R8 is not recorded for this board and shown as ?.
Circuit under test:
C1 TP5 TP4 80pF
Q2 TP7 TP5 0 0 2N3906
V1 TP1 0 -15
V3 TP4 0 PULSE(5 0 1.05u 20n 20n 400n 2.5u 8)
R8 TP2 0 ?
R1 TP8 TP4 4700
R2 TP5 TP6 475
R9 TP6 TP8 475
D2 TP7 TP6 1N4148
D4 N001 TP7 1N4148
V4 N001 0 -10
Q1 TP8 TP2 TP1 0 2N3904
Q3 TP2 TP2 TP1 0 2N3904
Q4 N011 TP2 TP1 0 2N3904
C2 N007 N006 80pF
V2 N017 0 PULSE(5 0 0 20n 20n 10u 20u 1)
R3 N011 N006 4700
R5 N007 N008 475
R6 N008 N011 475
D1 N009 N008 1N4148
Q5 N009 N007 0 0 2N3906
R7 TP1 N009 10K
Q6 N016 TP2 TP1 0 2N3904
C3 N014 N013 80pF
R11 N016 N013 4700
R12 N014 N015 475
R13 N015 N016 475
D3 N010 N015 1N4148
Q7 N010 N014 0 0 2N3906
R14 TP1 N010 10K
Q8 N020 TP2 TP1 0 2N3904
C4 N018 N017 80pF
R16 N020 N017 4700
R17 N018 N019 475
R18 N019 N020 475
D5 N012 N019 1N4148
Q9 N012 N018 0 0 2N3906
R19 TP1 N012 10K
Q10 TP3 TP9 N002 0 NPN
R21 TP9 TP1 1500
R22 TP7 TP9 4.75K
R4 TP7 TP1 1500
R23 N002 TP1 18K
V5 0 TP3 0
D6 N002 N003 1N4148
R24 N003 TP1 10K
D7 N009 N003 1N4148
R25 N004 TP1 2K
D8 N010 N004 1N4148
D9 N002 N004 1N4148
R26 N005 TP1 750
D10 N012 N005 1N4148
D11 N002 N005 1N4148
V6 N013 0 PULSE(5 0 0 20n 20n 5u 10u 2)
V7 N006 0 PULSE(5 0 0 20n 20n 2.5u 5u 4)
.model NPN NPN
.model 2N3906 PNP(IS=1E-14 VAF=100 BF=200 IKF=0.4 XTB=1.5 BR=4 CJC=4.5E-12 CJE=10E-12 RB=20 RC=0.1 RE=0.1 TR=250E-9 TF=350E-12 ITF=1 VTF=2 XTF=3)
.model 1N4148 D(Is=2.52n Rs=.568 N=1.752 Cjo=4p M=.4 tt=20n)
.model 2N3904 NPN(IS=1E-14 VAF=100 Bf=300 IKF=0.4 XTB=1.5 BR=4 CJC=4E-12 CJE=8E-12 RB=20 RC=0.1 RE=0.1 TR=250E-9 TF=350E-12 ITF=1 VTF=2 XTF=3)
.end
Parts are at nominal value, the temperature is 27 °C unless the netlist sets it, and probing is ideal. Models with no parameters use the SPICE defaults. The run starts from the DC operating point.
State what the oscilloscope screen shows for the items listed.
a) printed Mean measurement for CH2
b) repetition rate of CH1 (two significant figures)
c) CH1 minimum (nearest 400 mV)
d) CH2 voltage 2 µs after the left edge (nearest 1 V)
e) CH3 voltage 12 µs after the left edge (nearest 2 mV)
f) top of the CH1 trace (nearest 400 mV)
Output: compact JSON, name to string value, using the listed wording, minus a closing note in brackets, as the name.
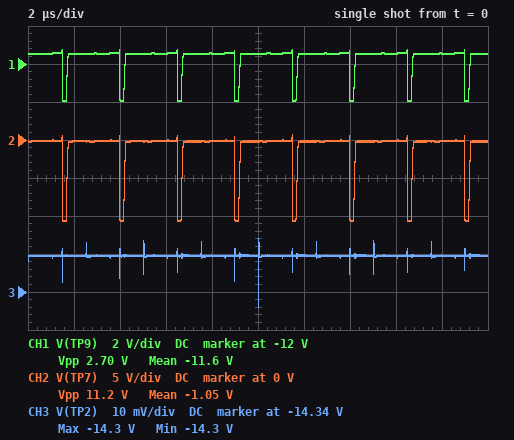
{"printed Mean measurement for CH2": "-1.05 V", "repetition rate of CH1": "400 kHz", "CH1 minimum": "-14.0 V", "CH2 voltage 2 µs after the left edge": "0 V", "CH3 voltage 12 µs after the left edge": "-14.330 V", "top of the CH1 trace": "-11.2 V"}
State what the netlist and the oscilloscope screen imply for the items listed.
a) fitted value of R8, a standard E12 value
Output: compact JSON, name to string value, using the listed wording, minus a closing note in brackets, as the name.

{"fitted value of R8, a standard E12 value": "8.2 kΩ"}
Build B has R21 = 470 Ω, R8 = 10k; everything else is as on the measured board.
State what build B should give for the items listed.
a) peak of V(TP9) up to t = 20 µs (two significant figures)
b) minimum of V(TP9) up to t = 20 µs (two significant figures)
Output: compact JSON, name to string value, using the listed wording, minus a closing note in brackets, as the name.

{"peak of V(TP9) up to t = 20 µs": "-14 V", "minimum of V(TP9) up to t = 20 µs": "-15 V"}
